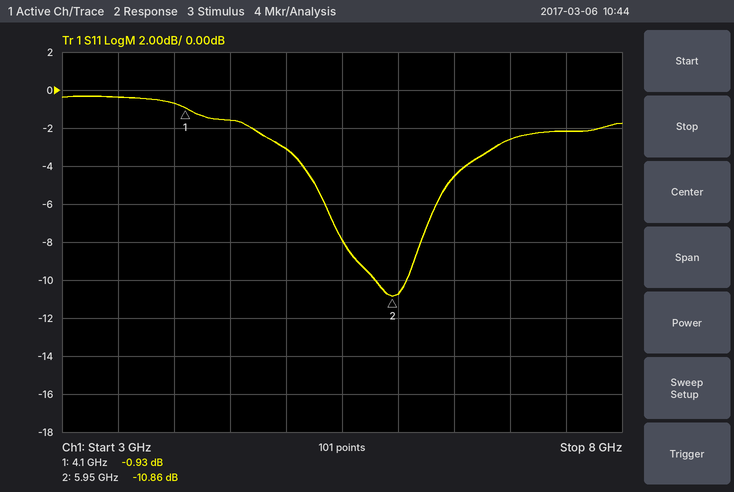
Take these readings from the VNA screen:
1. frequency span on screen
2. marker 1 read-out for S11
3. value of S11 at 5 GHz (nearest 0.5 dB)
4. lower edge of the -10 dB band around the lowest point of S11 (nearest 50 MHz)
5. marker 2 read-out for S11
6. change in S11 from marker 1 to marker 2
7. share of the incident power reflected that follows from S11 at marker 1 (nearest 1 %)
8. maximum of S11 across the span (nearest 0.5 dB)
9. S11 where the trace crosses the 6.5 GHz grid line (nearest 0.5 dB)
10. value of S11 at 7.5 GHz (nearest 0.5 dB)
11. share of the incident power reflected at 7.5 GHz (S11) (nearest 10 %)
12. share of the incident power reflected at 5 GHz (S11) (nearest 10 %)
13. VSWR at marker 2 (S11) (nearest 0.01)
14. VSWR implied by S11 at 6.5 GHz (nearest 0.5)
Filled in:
5 GHz
-0.93 dB
-3.0 dB
5.80 GHz
-10.86 dB
-9.93 dB
81 %
-0.5 dB
-4.5 dB
-2.0 dB
60 %
50 %
1.80
4.0
